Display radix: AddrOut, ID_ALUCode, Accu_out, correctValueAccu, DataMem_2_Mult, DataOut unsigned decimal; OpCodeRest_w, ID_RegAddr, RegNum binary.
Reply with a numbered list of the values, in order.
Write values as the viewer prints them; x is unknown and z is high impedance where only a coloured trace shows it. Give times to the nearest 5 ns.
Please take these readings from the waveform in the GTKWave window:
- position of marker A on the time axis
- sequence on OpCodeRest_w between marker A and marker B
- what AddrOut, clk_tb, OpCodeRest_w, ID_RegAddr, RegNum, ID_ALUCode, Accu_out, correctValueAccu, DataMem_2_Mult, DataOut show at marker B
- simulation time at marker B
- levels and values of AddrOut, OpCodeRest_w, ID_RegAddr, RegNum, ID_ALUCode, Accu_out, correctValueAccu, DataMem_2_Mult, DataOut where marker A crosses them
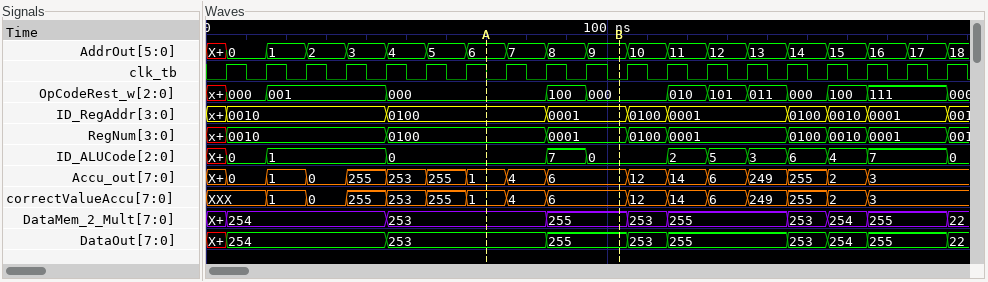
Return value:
1. 70 ns
2. 000, 100, 000
3. AddrOut=9, clk_tb=0, OpCodeRest_w=000, ID_RegAddr=0001, RegNum=0001, ID_ALUCode=0, Accu_out=6, correctValueAccu=6, DataMem_2_Mult=255, DataOut=255
4. 105 ns
5. AddrOut=6, OpCodeRest_w=000, ID_RegAddr=0100, RegNum=0100, ID_ALUCode=0, Accu_out=1, correctValueAccu=1, DataMem_2_Mult=253, DataOut=253
